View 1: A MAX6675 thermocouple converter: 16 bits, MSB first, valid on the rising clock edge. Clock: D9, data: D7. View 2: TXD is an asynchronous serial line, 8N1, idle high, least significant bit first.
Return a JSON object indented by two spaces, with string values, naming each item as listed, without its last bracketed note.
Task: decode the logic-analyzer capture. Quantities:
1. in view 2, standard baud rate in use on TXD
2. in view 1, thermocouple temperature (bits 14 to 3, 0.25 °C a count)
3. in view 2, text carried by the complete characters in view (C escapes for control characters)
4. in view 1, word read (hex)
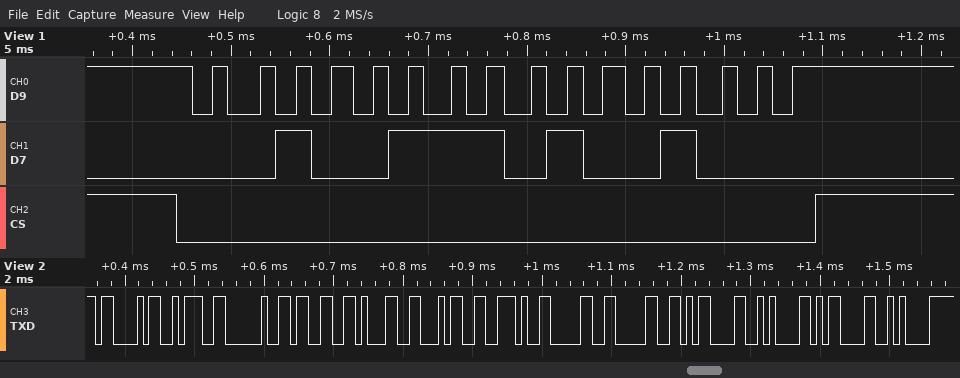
{
  "in view 2, standard baud rate in use on TXD": "115200 baud",
  "in view 1, thermocouple temperature": "314.25 °C",
  "in view 2, text carried by the complete characters in view": "\"C: 314.00\\r\\n\\r\\n\"",
  "in view 1, word read": "0x2748"
}
